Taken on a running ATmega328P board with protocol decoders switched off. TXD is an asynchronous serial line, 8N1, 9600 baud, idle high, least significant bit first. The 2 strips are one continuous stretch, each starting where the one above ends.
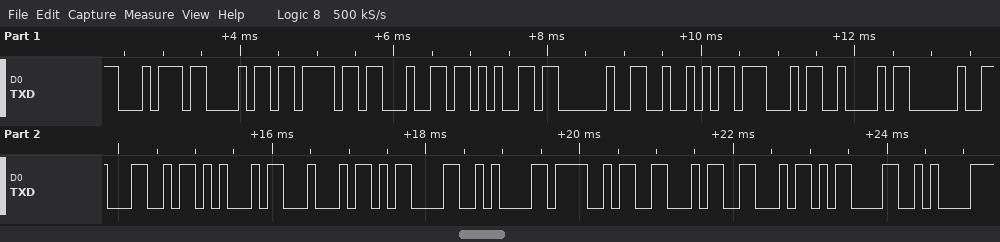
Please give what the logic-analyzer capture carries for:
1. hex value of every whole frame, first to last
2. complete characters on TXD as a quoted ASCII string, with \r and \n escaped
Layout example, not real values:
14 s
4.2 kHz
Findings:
74 68 6F 64 65 20 52 47 42 20 4C 45 44 0D 0A 4F 46 46 0D 0A
"thode RGB LED\r\nOFF\r\n"
